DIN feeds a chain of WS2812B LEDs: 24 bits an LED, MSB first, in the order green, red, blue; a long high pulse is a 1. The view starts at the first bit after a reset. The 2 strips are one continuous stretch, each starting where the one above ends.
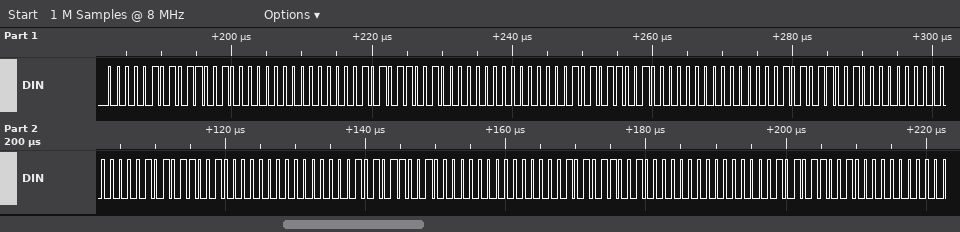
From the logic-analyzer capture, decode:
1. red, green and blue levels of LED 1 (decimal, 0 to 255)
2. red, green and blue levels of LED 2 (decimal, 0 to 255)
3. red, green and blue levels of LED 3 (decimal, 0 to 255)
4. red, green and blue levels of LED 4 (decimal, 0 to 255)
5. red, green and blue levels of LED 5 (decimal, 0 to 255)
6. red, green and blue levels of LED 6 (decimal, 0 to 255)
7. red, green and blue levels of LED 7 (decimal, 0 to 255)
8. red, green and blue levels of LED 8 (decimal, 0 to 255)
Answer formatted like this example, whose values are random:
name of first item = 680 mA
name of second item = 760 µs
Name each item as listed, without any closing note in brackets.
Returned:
red, green and blue levels of LED 1 = 100, 5, 0
red, green and blue levels of LED 2 = 100, 5, 0
red, green and blue levels of LED 3 = 100, 5, 0
red, green and blue levels of LED 4 = 100, 5, 0
red, green and blue levels of LED 5 = 100, 5, 0
red, green and blue levels of LED 6 = 100, 5, 0
red, green and blue levels of LED 7 = 100, 5, 0
red, green and blue levels of LED 8 = 100, 5, 0
